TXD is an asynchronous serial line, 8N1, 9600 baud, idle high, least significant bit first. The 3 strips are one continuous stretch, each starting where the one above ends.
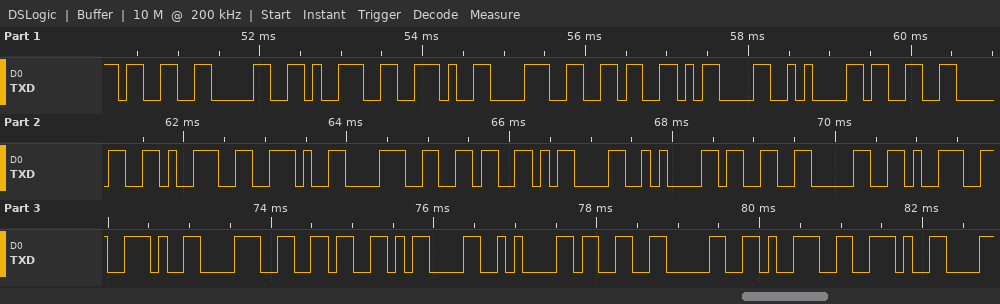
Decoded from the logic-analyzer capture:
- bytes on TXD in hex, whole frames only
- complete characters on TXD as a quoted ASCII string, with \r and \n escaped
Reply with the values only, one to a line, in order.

33 30 39 2E 38 36 0D 0A 33 30 39 2E 38 36 0D 0A 33 30 39 2E 38 36 0D 0A 33 30 39 2E
"309.86\r\n309.86\r\n309.86\r\n309."
